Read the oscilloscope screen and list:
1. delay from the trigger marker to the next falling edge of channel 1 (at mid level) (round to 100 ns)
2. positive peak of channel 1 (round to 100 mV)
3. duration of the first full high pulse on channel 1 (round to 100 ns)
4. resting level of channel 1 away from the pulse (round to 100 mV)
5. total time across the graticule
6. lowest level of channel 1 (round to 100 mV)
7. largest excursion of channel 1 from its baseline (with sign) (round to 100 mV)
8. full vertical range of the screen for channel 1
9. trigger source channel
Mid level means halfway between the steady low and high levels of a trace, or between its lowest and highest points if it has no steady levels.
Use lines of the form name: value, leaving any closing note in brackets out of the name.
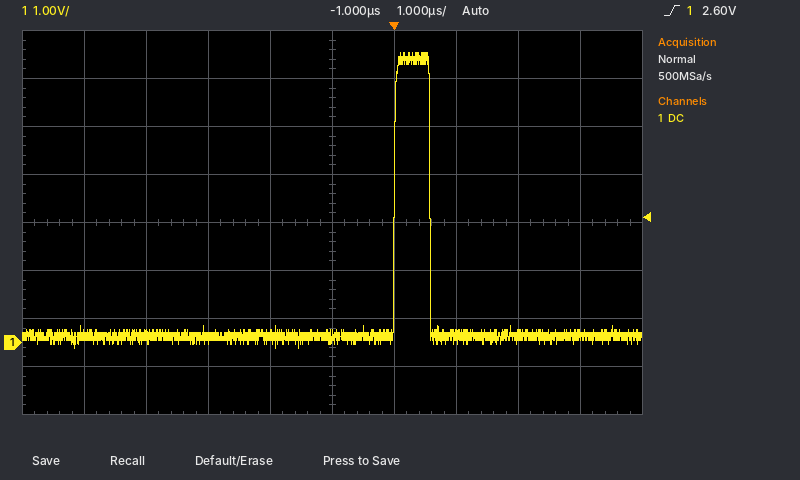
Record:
delay from the trigger marker to the next falling edge of channel 1 (at mid level): 600 ns
positive peak of channel 1: 6.0 V
duration of the first full high pulse on channel 1: 600 ns
resting level of channel 1 away from the pulse: 100 mV
total time across the graticule: 10 µs
lowest level of channel 1: -100 mV
largest excursion of channel 1 from its baseline (with sign): +5.9 V
full vertical range of the screen for channel 1: 8 V
trigger source channel: channel 1
